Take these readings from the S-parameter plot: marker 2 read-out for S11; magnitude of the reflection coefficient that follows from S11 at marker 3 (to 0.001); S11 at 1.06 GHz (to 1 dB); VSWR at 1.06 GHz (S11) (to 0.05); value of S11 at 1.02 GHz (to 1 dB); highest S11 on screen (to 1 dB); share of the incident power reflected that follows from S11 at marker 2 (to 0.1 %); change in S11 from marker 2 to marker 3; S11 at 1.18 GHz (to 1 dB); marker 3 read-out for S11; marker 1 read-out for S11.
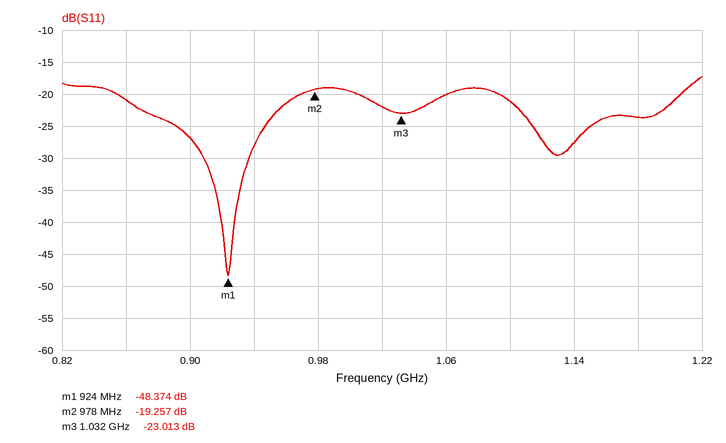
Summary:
-19.257 dB
0.071
-20 dB
1.20
-22 dB
-17 dB
1.2 %
-3.756 dB
-24 dB
-23.013 dB
-48.374 dB
